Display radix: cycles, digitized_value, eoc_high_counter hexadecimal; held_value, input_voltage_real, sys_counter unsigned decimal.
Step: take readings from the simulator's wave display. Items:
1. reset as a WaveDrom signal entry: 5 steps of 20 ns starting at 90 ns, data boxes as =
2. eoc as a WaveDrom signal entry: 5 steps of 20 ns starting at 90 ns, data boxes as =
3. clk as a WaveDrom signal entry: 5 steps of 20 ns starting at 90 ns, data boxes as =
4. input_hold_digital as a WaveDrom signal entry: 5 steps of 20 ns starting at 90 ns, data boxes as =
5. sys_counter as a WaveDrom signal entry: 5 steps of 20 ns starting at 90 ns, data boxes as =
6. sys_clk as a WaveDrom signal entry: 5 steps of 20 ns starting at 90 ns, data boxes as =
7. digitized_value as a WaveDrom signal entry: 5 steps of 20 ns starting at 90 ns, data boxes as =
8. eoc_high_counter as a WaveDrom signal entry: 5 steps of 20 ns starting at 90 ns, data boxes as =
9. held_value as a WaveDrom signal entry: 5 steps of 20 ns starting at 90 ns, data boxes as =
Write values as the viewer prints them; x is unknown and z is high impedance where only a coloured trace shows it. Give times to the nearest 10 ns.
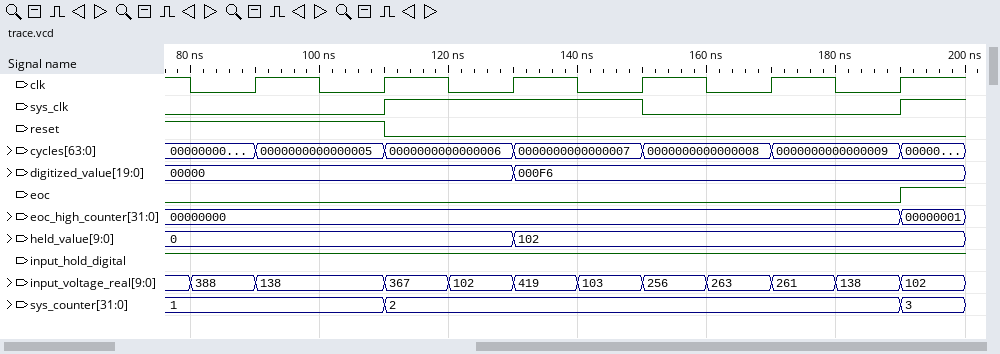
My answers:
{name: 'reset', wave: '10...'}
{name: 'eoc', wave: '0....'}
{name: 'clk', wave: 'p....'}
{name: 'input_hold_digital', wave: '1....'}
{name: 'sys_counter', wave: '==...', data: '1 2'}
{name: 'sys_clk', wave: '01.0.'}
{name: 'digitized_value', wave: '=.=..', data: '00000 000F6'}
{name: 'eoc_high_counter', wave: '=....', data: '00000000'}
{name: 'held_value', wave: '=.=..', data: '0 102'}
